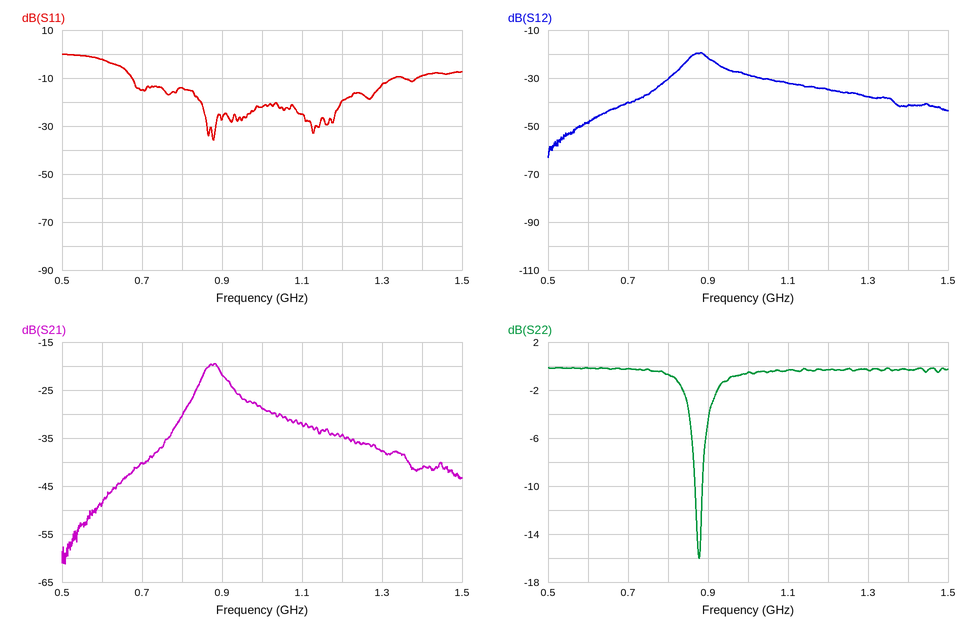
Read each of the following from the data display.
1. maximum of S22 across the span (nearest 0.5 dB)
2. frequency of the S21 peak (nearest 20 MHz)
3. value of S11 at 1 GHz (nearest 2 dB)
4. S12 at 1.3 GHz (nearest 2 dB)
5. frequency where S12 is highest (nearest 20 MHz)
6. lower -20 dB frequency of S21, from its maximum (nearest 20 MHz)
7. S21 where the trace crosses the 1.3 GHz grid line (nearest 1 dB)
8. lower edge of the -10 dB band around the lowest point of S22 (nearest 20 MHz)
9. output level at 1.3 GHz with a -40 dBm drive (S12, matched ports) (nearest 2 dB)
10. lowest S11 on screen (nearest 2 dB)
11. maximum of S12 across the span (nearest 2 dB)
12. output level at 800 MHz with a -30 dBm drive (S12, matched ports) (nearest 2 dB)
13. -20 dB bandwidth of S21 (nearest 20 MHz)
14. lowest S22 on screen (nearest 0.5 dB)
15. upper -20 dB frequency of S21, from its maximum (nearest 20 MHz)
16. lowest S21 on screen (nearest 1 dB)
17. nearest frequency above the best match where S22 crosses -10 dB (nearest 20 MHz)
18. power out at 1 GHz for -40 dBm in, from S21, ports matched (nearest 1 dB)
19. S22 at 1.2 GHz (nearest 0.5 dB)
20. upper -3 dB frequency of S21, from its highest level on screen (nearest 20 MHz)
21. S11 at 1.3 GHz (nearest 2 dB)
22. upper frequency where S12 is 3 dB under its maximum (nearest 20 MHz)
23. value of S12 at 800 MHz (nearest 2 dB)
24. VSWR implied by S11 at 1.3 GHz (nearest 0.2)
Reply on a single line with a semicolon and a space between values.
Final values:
0.0 dB; 880 MHz; -22 dB; -38 dB; 880 MHz; 720 MHz; -38 dB; 860 MHz; -78 dBm; -36 dB; -20 dB; -60 dBm; 640 MHz; -16.0 dB; 1.36 GHz; -61 dB; 880 MHz; -69 dBm; -0.5 dB; 900 MHz; -12 dB; 900 MHz; -30 dB; 1.6
